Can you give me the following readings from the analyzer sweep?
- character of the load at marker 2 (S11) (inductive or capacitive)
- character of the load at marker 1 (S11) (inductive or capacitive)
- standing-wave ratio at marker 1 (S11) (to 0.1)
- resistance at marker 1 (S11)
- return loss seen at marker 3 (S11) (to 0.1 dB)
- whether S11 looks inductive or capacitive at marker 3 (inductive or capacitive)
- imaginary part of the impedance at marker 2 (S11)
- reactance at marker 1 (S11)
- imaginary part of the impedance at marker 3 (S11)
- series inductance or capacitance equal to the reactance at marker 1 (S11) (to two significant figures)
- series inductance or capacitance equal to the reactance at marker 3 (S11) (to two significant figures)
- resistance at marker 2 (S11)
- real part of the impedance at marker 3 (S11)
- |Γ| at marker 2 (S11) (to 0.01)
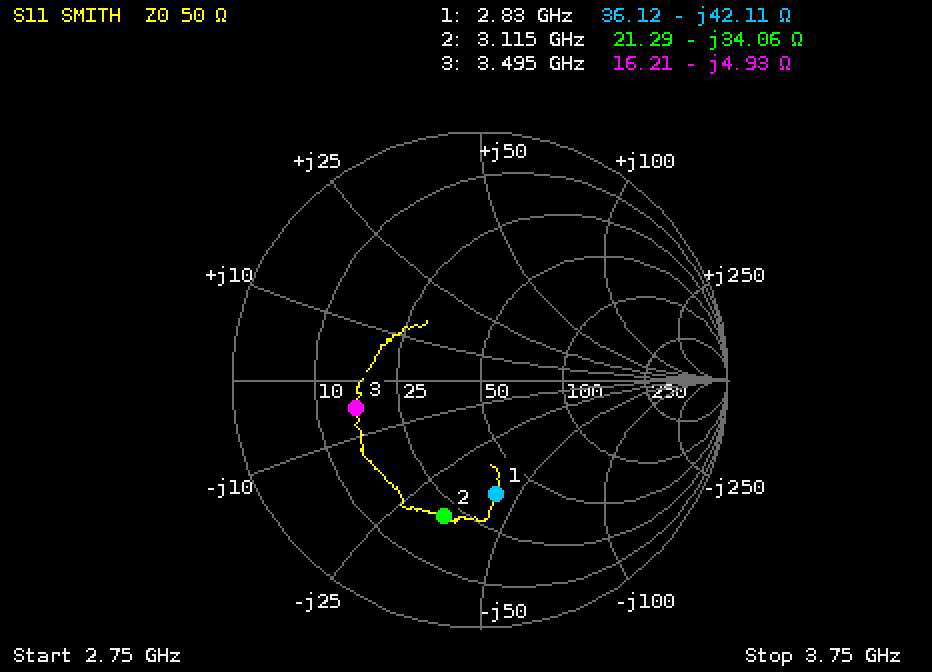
capacitive
capacitive
2.7
36.12 Ω
5.8 dB
capacitive
-34.06 Ω
-42.11 Ω
-4.93 Ω
1.3 pF
9.2 pF
21.29 Ω
16.21 Ω
0.56
